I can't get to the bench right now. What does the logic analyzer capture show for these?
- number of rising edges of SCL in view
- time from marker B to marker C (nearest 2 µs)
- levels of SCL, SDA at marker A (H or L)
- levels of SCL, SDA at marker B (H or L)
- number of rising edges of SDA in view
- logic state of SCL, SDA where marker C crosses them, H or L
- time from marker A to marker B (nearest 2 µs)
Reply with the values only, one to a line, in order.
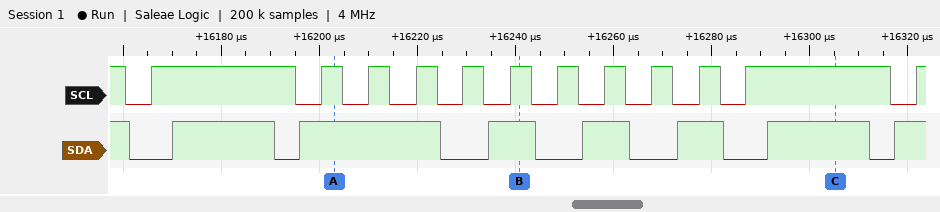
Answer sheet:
12
64 µs
SCL=H, SDA=H
SCL=H, SDA=H
7
SCL=H, SDA=H
38 µs
